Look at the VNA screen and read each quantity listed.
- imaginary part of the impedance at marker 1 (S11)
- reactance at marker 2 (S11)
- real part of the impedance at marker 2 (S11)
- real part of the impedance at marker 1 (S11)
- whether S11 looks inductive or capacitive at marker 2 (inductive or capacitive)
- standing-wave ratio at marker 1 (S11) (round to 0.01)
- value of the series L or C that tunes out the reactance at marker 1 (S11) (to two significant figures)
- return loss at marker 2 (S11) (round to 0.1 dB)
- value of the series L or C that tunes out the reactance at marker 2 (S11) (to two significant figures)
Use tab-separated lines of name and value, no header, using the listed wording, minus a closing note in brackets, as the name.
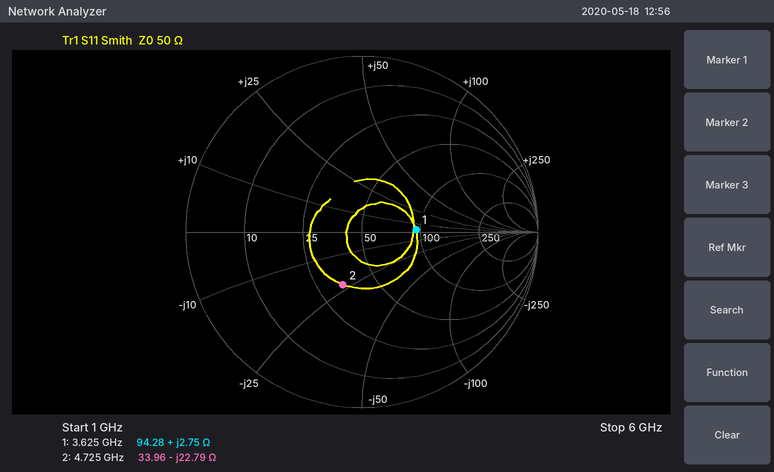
imaginary part of the impedance at marker 1	+2.75 Ω
reactance at marker 2	-22.79 Ω
real part of the impedance at marker 2	33.96 Ω
real part of the impedance at marker 1	94.28 Ω
whether S11 looks inductive or capacitive at marker 2	capacitive
standing-wave ratio at marker 1 (S11)	1.89
value of the series L or C that tunes out the reactance at marker 1 (S11)	16 pF
return loss at marker 2 (S11)	9.9 dB
value of the series L or C that tunes out the reactance at marker 2 (S11)	770 pH
